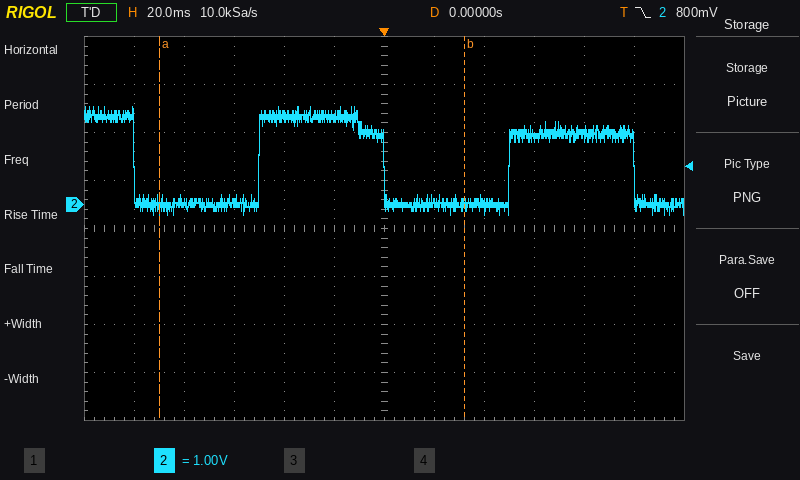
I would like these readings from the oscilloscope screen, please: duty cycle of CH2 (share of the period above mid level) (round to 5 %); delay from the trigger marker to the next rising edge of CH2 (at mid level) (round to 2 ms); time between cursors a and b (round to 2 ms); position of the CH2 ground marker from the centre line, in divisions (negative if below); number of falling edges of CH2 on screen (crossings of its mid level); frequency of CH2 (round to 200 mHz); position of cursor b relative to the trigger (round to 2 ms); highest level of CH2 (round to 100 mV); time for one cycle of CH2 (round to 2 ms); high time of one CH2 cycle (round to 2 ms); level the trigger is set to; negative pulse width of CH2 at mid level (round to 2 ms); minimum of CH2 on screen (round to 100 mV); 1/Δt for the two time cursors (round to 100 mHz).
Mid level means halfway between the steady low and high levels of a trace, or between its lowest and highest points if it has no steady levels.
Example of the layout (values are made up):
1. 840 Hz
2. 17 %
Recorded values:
1. 50 %
2. 50 ms
3. 122 ms
4. +0.5 div
5. 3
6. 10.0 Hz
7. +32 ms
8. 2.0 V
9. 100 ms
10. 50 ms
11. 800 mV
12. 50 ms
13. -200 mV
14. 8.2 Hz
